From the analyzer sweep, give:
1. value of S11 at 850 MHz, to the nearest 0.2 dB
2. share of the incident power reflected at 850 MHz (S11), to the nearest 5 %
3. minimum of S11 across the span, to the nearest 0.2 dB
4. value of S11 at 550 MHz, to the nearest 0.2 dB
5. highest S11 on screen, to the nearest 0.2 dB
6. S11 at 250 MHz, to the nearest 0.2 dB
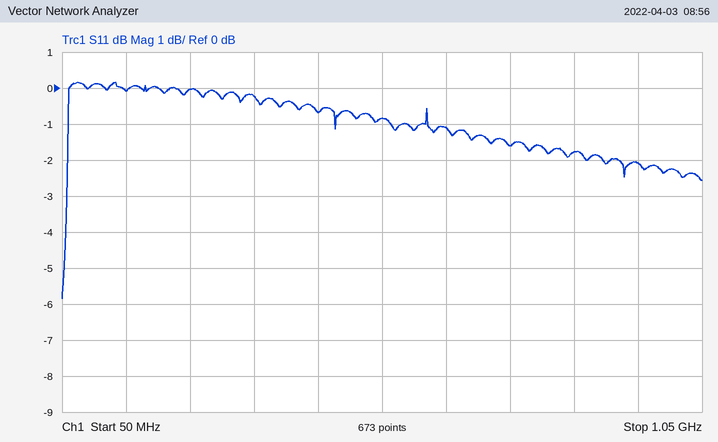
-1.8 dB
65 %
-5.8 dB
-0.8 dB
0.2 dB
0.0 dB
